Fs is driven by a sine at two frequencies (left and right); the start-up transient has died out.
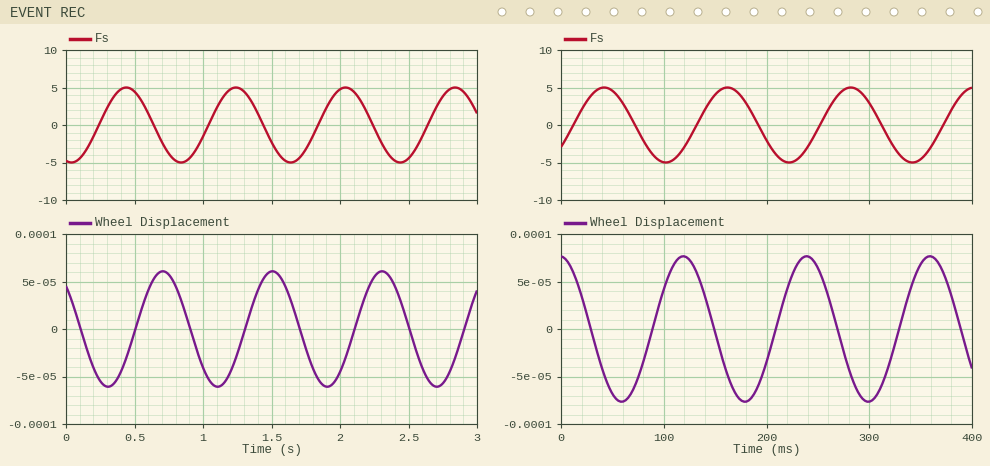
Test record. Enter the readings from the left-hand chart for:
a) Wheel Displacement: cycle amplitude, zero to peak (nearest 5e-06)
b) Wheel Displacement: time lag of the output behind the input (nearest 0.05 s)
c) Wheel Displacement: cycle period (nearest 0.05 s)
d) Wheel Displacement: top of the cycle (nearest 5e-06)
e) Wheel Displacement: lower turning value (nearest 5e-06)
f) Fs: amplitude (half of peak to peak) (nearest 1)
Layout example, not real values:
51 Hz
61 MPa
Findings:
0.000060
0.25 s
0.80 s
0.000060
-0.000060
5
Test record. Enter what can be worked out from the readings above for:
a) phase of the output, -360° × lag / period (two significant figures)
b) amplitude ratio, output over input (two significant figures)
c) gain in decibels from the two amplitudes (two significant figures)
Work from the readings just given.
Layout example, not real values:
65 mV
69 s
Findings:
-110°
0.000012
-98 dB
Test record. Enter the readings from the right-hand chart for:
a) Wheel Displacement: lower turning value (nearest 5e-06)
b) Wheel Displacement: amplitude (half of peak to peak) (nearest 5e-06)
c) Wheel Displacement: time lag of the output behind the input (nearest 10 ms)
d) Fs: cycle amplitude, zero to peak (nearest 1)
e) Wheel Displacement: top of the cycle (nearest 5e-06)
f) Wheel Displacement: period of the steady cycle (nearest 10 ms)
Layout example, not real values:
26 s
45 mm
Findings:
-0.000075
0.000075
80 ms
5
0.000075
120 ms
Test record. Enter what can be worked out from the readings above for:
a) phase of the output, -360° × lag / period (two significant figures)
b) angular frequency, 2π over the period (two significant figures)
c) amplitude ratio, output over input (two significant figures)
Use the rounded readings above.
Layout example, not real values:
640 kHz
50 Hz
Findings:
-240°
0.052 rad/ms
0.000015
